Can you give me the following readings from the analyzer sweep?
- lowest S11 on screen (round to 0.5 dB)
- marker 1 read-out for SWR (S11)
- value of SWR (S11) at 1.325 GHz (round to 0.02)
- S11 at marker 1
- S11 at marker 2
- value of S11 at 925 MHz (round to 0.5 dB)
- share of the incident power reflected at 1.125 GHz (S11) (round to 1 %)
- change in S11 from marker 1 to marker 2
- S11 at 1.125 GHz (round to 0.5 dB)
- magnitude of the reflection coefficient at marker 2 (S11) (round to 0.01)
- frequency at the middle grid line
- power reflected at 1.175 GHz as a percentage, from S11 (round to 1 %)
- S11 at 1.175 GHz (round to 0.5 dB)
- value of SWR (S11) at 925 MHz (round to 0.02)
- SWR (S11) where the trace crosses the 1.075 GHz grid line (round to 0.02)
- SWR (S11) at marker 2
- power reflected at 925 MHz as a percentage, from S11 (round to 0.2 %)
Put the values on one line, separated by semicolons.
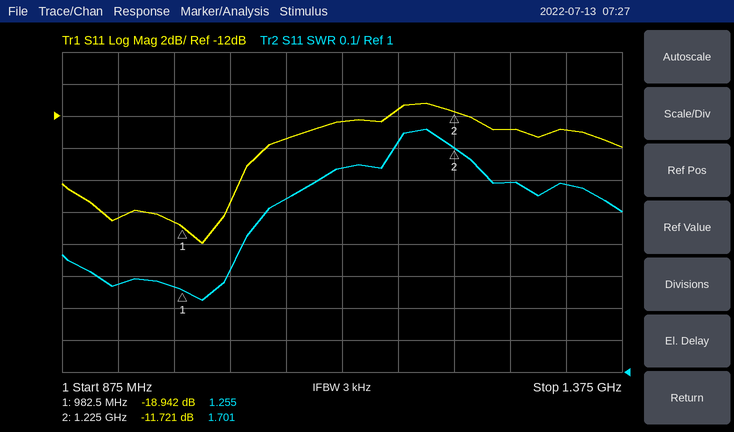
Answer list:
-20.0 dB; 1.255; 1.58; -18.942 dB; -11.721 dB; -18.5 dB; 6 %; 7.221 dB; -12.5 dB; 0.26; 1.125 GHz; 7 %; -11.5 dB; 1.28; 1.54; 1.701; 1.4 %
